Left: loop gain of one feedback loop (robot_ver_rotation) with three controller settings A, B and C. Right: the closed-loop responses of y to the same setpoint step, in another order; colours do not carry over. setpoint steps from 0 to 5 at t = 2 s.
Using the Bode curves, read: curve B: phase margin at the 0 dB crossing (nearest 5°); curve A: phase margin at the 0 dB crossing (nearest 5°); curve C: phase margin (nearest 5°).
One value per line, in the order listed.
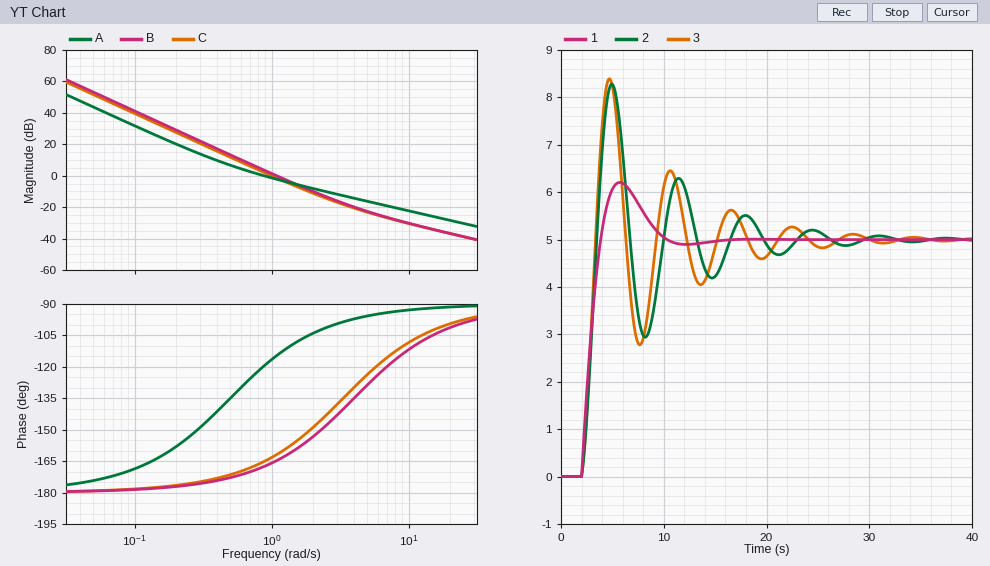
15°
60°
15°
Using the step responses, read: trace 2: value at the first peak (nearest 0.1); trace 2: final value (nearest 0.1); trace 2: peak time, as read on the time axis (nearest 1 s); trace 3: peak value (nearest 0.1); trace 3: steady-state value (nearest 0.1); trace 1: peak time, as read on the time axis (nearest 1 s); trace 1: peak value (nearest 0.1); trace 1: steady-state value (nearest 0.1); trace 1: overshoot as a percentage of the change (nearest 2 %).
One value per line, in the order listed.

8.3
5.0
5 s
8.4
5.0
6 s
6.2
5.0
24 %
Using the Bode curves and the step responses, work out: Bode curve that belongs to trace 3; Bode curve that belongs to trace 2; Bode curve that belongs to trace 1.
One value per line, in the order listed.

B
C
A
